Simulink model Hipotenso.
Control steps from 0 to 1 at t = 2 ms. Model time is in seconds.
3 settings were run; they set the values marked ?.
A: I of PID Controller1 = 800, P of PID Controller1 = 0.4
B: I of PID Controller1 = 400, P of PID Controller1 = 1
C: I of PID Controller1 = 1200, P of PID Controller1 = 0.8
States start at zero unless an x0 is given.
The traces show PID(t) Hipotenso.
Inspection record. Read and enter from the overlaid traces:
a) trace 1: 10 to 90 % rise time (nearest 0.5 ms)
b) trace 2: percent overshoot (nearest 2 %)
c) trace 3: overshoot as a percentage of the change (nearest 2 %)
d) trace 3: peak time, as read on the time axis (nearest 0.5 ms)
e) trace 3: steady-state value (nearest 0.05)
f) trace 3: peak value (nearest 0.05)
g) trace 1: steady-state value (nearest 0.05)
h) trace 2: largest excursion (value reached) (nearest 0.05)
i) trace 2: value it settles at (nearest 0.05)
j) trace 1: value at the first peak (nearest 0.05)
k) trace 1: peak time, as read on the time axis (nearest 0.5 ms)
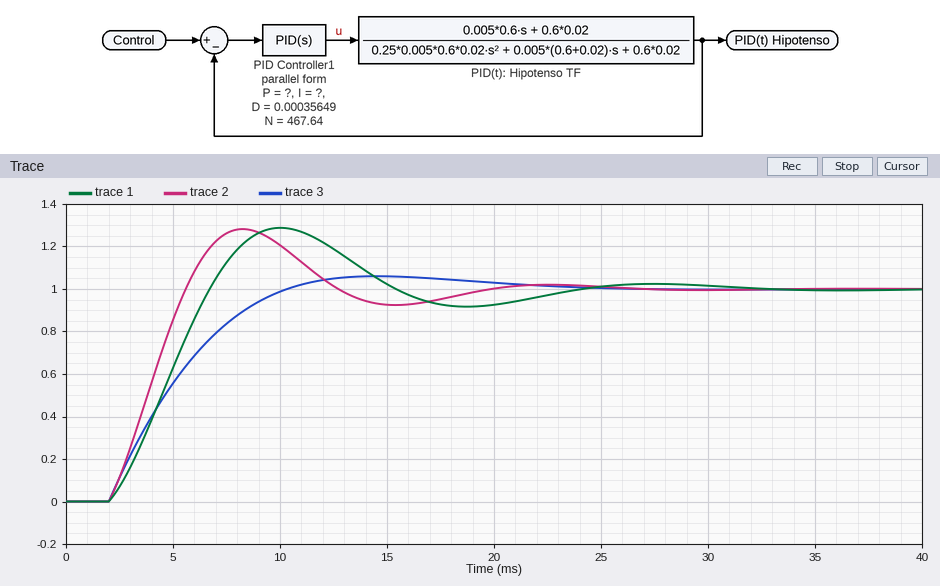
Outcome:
3.5 ms
28 %
6 %
14.5 ms
1.00
1.05
1.00
1.30
1.00
1.30
10.0 ms
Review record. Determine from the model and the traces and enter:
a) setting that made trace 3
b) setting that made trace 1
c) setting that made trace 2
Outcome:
B
A
C
